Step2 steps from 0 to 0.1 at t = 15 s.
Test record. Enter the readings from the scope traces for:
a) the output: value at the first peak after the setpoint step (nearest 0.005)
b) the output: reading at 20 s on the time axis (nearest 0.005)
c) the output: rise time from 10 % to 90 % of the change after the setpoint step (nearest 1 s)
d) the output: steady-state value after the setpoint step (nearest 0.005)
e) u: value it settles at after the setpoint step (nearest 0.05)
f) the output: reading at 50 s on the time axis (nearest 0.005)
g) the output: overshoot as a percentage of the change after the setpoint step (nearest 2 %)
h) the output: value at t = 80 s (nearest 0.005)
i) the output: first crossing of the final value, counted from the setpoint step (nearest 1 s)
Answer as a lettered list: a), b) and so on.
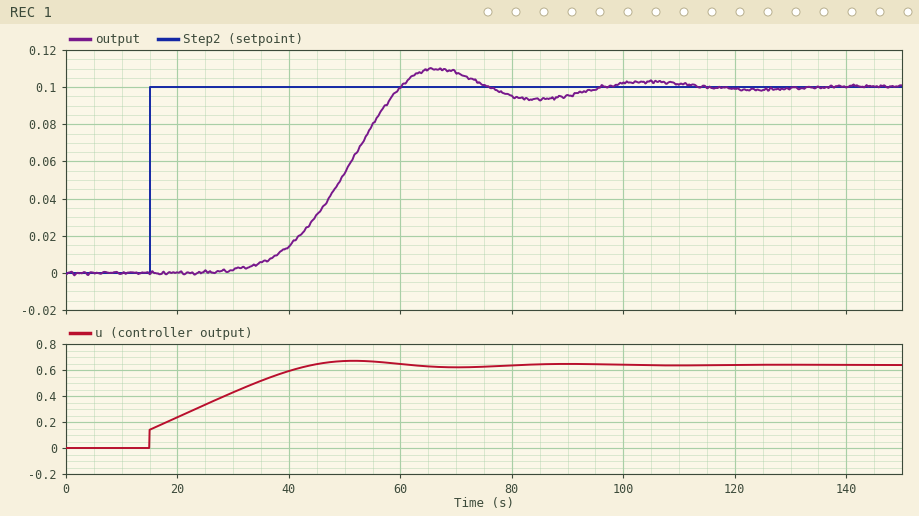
a) 0.110
b) 0.000
c) 19 s
d) 0.100
e) 0.65
f) 0.055
g) 10 %
h) 0.095
i) 45 s
